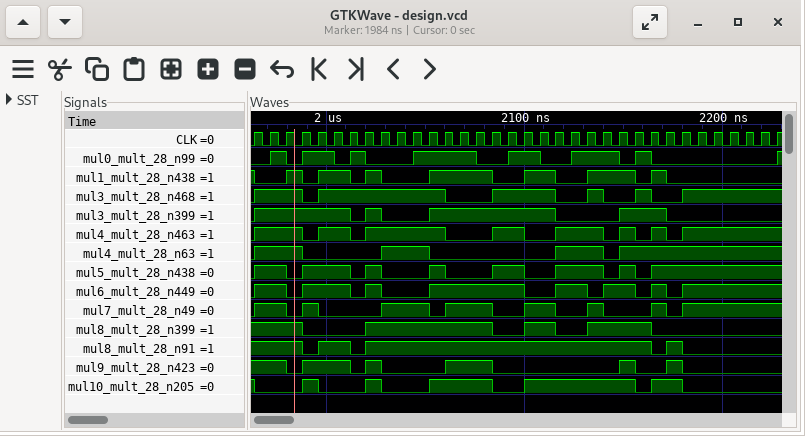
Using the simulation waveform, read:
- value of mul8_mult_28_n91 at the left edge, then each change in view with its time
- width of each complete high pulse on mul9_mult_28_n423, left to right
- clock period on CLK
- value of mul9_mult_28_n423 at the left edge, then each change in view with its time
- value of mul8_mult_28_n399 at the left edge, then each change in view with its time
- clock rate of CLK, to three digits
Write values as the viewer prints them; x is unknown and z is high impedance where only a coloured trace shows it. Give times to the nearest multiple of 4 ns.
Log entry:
1, 0 at 1988 ns, 1 at 1996 ns, 0 at 2012 ns, 1 at 2020 ns, 0 at 2164 ns, 1 at 2172 ns, 0 at 2180 ns
24 ns, 8 ns, 24 ns, 8 ns, 8 ns
8 ns
1, 0 at 1980 ns, 1 at 1988 ns, 0 at 2012 ns, 1 at 2020 ns, 0 at 2028 ns, 1 at 2060 ns, 0 at 2084 ns, 1 at 2148 ns, 0 at 2156 ns, 1 at 2172 ns, 0 at 2180 ns
1, 0 at 1988 ns, 1 at 2020 ns, 0 at 2084 ns, 1 at 2100 ns, 0 at 2116 ns, 1 at 2132 ns, 0 at 2164 ns
125 MHz
